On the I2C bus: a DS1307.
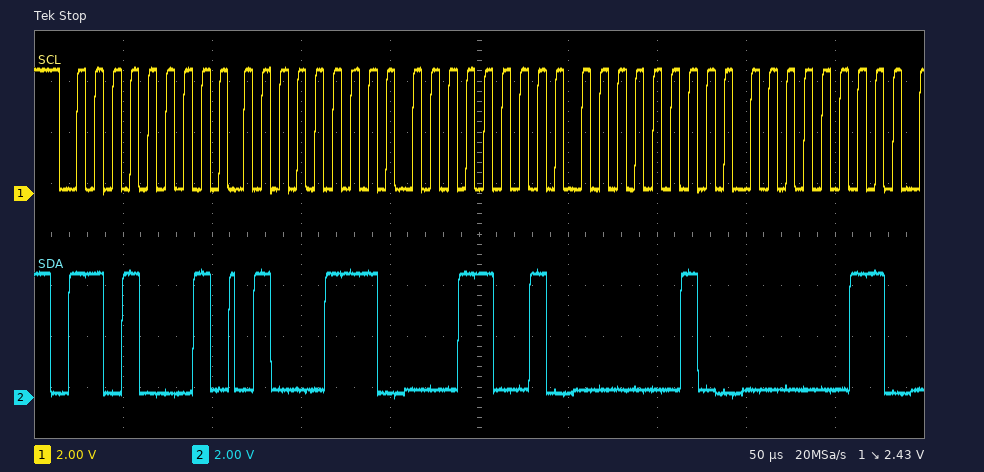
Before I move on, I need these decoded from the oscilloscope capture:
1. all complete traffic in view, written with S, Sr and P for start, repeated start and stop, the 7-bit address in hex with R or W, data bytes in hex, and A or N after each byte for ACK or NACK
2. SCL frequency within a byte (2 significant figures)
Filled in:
S 68R A 47 A 19 A 02 A 03 A
100 kHz
